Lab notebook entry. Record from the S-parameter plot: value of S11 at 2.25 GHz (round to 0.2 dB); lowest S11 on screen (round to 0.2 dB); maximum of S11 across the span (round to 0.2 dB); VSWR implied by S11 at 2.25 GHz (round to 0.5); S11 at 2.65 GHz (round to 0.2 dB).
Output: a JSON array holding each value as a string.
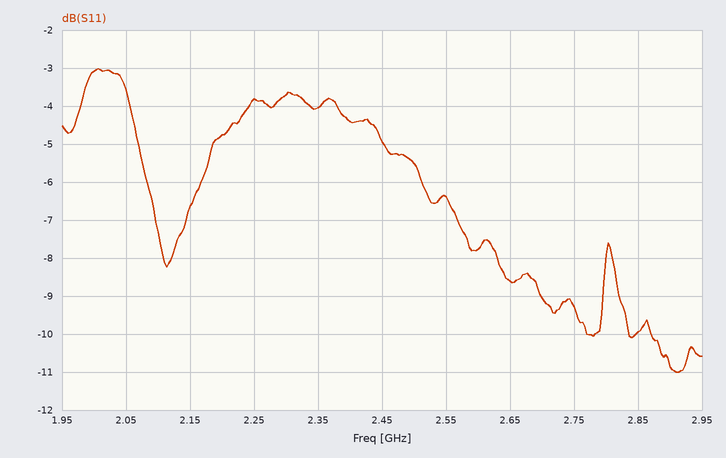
["-3.8 dB", "-11.0 dB", "-3.0 dB", "4.5", "-8.6 dB"]
